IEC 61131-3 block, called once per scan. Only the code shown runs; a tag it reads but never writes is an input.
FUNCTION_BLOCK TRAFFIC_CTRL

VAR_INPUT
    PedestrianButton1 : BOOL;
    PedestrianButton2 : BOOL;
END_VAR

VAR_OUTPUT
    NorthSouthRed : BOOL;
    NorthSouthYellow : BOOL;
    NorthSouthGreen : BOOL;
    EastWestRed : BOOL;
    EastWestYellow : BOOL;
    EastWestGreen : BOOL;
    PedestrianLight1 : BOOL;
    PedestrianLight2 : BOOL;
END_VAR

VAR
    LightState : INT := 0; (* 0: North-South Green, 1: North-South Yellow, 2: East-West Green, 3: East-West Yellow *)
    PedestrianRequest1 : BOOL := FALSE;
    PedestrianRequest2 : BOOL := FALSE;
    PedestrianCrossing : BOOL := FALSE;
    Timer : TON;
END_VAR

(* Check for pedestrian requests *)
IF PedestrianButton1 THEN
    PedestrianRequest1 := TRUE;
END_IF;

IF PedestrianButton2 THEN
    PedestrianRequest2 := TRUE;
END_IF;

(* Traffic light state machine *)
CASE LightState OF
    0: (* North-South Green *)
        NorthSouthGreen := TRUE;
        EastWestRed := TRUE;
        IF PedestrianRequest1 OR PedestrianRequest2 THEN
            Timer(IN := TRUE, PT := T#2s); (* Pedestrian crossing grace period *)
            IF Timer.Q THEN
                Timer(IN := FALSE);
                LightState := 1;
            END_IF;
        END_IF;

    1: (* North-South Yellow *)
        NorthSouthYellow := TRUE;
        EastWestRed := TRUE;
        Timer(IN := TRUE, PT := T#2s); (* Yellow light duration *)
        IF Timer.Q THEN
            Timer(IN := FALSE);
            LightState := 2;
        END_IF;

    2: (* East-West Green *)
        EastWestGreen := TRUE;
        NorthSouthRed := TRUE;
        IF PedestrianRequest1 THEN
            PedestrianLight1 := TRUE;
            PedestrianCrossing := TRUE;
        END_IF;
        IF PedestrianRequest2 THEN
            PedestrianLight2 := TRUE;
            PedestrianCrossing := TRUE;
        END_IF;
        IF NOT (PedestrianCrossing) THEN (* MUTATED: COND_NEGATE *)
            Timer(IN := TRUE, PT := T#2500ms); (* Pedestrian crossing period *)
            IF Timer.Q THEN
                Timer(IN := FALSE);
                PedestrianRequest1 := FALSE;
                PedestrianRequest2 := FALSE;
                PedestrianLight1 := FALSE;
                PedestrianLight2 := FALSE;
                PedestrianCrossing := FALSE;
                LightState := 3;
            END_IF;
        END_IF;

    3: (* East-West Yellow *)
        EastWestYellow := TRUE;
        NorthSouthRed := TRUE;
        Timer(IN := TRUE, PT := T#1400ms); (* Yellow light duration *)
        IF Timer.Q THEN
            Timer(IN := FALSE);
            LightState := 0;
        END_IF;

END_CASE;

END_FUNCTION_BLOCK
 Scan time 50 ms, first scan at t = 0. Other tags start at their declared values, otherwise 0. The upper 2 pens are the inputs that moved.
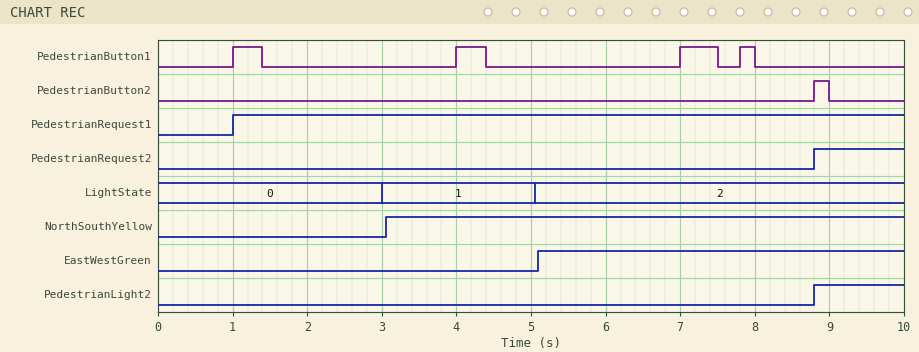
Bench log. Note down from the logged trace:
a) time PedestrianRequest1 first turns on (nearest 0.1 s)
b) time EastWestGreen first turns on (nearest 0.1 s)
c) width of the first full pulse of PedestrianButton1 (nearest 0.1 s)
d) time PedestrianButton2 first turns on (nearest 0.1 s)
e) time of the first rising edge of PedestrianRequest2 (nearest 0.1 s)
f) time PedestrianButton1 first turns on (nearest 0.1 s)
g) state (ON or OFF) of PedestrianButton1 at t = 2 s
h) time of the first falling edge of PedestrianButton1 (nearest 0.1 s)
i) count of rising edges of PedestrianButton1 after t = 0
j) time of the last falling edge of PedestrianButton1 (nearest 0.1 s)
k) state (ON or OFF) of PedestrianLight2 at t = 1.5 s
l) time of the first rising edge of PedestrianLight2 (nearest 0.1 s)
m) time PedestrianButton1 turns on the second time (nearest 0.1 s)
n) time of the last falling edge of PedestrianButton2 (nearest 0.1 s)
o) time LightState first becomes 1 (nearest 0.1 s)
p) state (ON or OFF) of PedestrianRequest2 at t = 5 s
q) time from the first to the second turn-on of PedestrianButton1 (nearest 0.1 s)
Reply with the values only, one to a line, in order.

1.0 s
5.1 s
0.4 s
8.8 s
8.8 s
1.0 s
OFF
1.4 s
4
8.0 s
OFF
8.8 s
4.0 s
9.0 s
3.0 s
OFF
3.0 s
